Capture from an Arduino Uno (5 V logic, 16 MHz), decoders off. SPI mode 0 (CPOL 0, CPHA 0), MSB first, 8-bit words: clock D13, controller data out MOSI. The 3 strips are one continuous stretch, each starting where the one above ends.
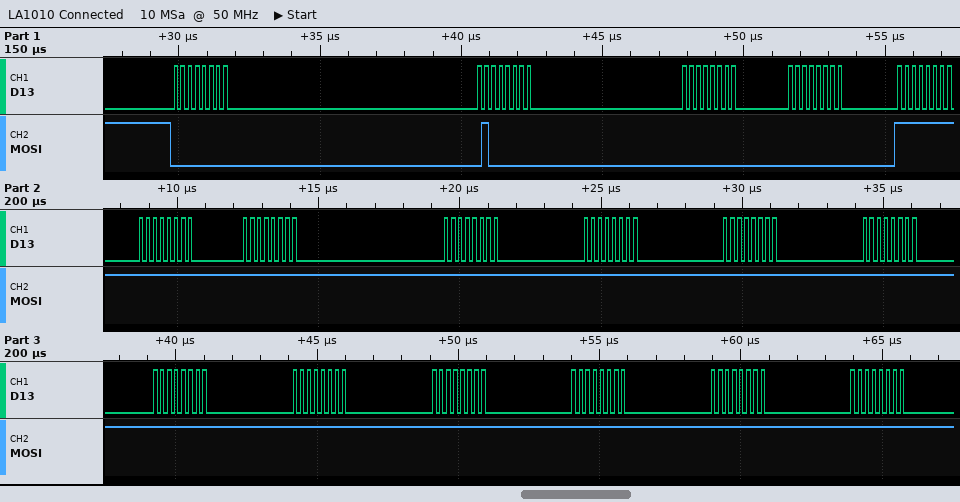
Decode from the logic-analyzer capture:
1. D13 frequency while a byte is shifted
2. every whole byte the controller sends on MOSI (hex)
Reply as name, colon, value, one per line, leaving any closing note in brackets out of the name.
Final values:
D13 frequency while a byte is shifted: 4 MHz
every whole byte the controller sends on MOSI: 00 40 00 00 FF FF FF FF FF FF FF FF FF FF FF FF FF
